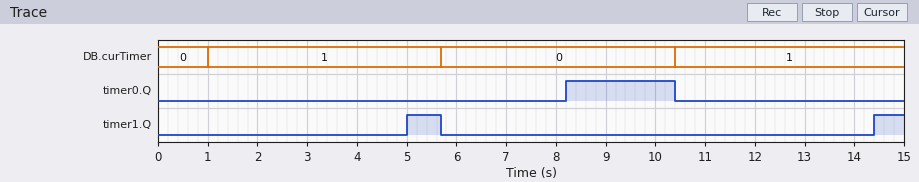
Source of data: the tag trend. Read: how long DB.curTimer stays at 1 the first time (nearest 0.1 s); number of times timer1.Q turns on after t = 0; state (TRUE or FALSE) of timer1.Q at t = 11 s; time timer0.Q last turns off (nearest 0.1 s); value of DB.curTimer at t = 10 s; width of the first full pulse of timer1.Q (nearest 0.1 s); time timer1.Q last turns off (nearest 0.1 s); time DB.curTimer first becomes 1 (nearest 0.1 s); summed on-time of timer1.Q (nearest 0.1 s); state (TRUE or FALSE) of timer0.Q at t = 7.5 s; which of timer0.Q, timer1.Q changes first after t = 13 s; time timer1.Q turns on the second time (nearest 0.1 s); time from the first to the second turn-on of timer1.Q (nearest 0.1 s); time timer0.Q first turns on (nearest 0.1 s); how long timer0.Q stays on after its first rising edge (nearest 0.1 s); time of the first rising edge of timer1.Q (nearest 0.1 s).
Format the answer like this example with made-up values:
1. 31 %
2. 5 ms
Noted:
1. 4.7 s
2. 2
3. FALSE
4. 10.4 s
5. 0
6. 0.7 s
7. 5.7 s
8. 1.0 s
9. 1.3 s
10. FALSE
11. timer1.Q
12. 14.4 s
13. 9.4 s
14. 8.2 s
15. 2.2 s
16. 5.0 s
